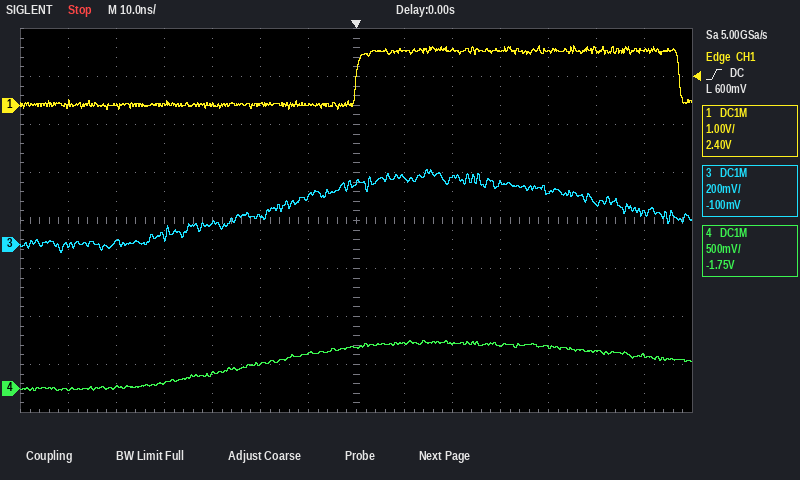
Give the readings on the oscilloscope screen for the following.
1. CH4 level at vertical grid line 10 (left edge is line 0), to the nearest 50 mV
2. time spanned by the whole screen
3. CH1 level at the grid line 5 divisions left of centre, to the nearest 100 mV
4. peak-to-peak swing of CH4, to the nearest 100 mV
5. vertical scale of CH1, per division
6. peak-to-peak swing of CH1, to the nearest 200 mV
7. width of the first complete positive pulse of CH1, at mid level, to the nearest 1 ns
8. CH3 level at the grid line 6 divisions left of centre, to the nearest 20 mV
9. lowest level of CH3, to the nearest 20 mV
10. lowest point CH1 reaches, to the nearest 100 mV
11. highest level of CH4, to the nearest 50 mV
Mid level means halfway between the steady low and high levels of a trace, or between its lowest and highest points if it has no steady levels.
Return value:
450 mV
140 ns
0.0 V
500 mV
1 V
1.4 V
67 ns
0 mV
-40 mV
-100 mV
500 mV
